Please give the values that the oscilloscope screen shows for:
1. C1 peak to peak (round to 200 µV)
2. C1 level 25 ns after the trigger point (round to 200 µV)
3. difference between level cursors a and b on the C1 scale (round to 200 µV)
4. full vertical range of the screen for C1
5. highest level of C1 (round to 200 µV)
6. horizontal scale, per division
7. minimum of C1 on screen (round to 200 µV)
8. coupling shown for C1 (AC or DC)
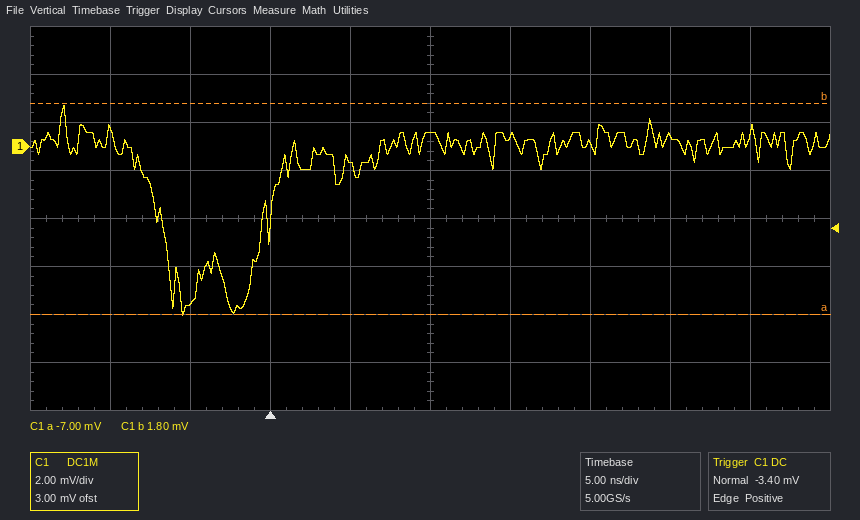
8.8 mV
400 µV
8.8 mV
16 mV
1.8 mV
5 ns
-7.0 mV
DC
